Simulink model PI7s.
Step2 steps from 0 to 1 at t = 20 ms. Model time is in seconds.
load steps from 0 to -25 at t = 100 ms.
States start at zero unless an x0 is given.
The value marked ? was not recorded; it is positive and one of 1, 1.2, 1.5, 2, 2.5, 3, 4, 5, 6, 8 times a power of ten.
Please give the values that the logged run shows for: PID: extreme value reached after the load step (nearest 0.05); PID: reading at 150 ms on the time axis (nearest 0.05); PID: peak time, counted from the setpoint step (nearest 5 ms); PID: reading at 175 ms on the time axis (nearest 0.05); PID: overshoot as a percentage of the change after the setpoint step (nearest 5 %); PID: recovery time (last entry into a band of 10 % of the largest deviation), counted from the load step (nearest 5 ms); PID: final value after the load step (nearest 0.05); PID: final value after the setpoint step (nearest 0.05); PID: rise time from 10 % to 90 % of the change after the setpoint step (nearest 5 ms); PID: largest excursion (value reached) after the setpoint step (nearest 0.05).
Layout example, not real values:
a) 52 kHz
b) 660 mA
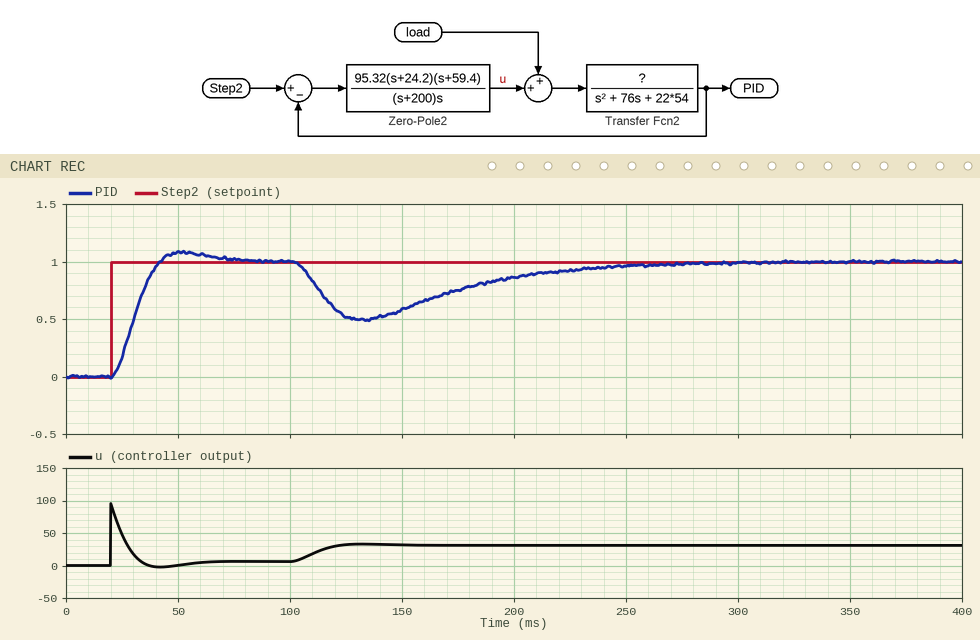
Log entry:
a) 0.50
b) 0.60
c) 30 ms
d) 0.75
e) 10 %
f) 140 ms
g) 1.00
h) 1.00
i) 15 ms
j) 1.10
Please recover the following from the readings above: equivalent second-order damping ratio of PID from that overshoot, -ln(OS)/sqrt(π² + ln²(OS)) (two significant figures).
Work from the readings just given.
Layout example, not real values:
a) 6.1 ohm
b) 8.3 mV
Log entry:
a) 0.59
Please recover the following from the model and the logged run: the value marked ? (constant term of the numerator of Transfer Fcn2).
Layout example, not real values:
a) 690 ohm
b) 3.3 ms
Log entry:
a) 200
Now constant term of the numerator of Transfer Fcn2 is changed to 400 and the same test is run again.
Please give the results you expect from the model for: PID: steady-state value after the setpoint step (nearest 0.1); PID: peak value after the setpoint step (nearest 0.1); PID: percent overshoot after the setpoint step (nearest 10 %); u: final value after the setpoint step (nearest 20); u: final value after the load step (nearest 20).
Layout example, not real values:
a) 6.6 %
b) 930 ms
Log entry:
a) 1.0
b) 1.2
c) 20 %
d) 0
e) 20
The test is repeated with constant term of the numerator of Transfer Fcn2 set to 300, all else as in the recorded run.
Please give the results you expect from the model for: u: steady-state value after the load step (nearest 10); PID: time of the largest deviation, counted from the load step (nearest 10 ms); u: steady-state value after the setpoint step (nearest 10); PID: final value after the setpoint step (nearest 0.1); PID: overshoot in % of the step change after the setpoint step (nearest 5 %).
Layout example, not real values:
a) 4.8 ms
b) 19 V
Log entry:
a) 30
b) 30 ms
c) 0
d) 1.0
e) 15 %
